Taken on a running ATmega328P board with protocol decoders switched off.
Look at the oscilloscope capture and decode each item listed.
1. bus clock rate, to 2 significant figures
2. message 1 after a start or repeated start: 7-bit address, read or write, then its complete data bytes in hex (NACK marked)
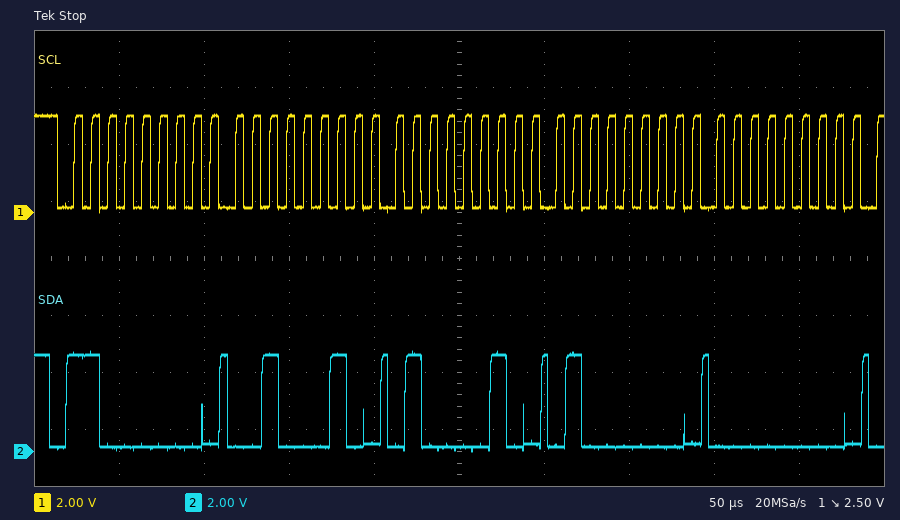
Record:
100 kHz
0x60 write: 22 42 40 00
